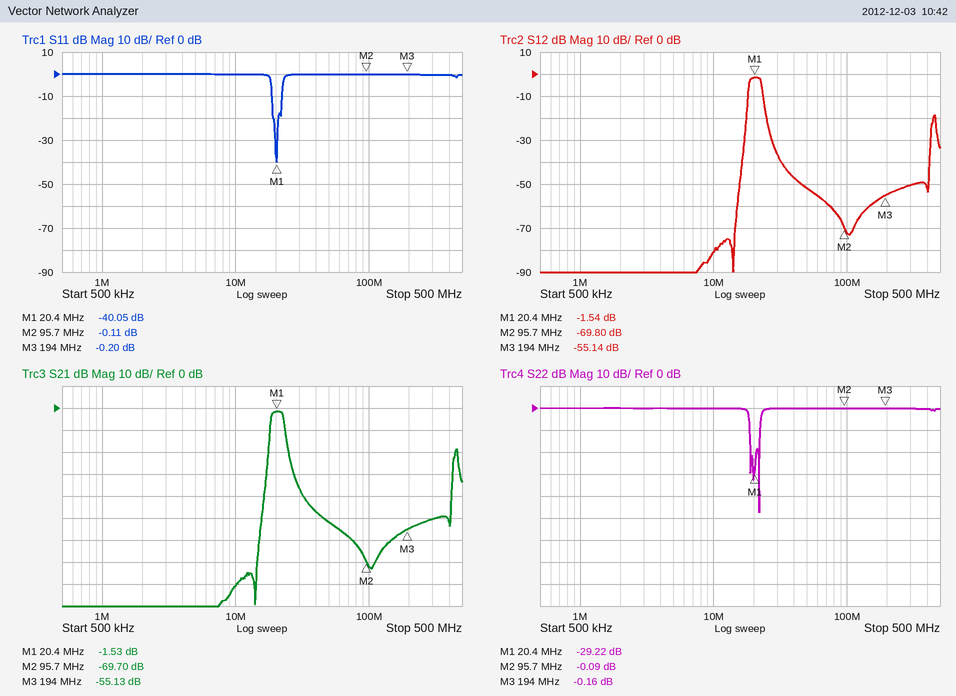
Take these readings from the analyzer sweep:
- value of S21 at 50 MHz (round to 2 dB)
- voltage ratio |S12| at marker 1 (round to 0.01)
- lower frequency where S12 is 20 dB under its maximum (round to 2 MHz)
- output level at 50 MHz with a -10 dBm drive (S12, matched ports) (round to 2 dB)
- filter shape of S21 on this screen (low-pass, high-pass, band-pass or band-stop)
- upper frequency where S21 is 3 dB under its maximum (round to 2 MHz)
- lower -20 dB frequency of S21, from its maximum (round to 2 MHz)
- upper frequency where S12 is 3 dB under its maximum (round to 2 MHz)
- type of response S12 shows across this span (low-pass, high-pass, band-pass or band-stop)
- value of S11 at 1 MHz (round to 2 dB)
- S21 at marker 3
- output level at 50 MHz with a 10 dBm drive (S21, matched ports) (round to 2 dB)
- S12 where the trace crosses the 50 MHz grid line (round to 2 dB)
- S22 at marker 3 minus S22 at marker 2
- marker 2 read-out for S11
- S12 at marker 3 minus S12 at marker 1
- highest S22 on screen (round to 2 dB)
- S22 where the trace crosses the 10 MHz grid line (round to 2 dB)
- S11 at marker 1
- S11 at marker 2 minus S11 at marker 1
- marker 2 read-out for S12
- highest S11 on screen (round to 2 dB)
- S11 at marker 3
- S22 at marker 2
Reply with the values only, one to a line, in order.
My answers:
-52 dB
0.84
18 MHz
-62 dBm
band-pass
22 MHz
18 MHz
22 MHz
band-pass
0 dB
-55.13 dB
-42 dBm
-52 dB
-0.07 dB
-0.11 dB
-53.60 dB
0 dB
0 dB
-40.05 dB
39.94 dB
-69.80 dB
0 dB
-0.20 dB
-0.09 dB
